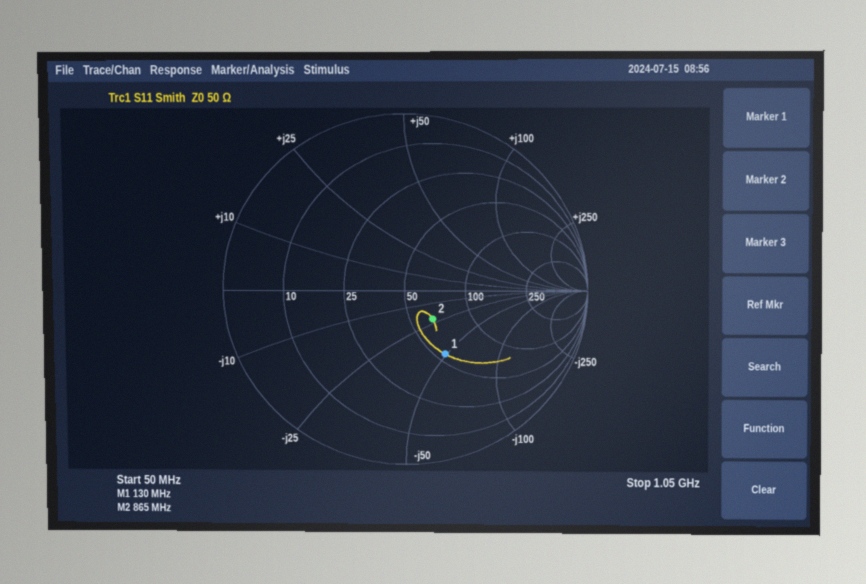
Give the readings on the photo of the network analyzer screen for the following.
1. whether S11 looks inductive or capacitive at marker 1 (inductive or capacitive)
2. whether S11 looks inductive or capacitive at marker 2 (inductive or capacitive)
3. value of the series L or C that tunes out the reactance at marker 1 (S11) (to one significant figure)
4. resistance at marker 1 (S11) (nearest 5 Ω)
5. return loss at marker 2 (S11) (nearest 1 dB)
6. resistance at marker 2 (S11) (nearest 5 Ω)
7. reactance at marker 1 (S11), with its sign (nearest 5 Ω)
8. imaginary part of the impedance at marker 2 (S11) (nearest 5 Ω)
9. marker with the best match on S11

capacitive
capacitive
60 nH
55 Ω
13 dB
65 Ω
-50 Ω
-20 Ω
marker 2
